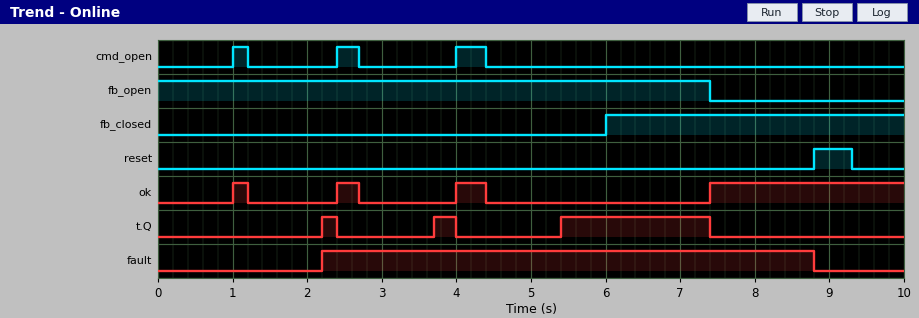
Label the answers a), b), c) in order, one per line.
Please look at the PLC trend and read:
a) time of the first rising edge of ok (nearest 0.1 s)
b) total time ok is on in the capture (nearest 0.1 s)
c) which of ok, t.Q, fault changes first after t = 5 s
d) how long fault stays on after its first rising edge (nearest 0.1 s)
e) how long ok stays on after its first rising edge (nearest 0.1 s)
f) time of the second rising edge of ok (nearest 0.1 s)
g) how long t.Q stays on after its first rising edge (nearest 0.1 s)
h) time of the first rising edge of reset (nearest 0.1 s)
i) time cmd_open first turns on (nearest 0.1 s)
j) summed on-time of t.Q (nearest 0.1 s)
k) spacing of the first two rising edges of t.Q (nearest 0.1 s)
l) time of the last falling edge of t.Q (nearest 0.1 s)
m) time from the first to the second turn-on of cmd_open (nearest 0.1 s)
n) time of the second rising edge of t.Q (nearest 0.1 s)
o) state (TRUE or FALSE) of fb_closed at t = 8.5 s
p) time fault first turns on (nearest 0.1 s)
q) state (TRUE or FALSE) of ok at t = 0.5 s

a) 1.0 s
b) 3.5 s
c) t.Q
d) 6.6 s
e) 0.2 s
f) 2.4 s
g) 0.2 s
h) 8.8 s
i) 1.0 s
j) 2.5 s
k) 1.5 s
l) 7.4 s
m) 1.4 s
n) 3.7 s
o) TRUE
p) 2.2 s
q) FALSE
